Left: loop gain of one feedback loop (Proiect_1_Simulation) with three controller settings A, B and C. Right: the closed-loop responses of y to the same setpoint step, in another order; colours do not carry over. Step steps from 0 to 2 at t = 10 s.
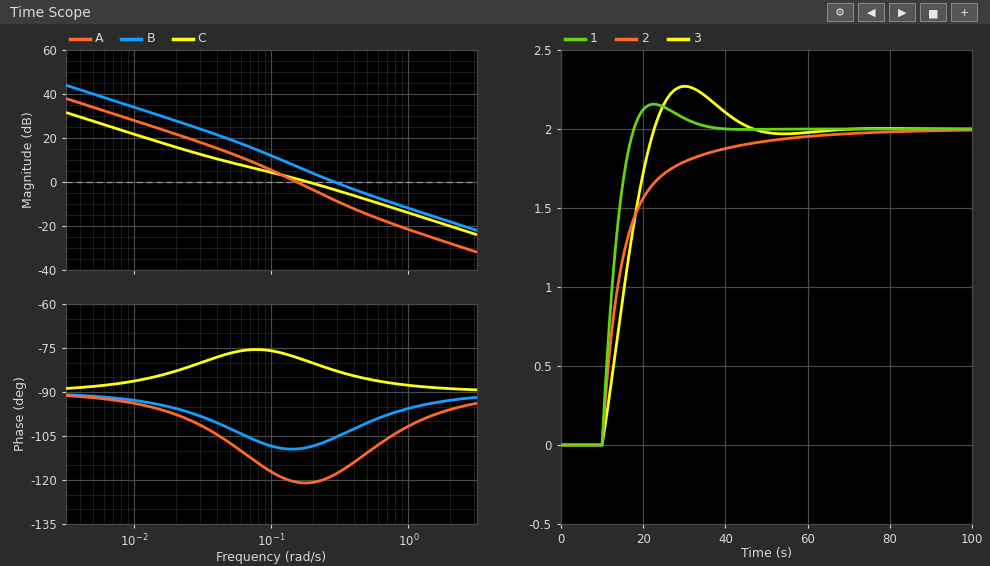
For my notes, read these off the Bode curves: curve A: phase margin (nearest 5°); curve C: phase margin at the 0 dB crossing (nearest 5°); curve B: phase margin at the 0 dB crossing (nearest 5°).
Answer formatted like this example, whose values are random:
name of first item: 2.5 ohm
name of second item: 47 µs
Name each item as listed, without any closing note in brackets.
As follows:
curve A: phase margin: 60°
curve C: phase margin at the 0 dB crossing: 100°
curve B: phase margin at the 0 dB crossing: 75°
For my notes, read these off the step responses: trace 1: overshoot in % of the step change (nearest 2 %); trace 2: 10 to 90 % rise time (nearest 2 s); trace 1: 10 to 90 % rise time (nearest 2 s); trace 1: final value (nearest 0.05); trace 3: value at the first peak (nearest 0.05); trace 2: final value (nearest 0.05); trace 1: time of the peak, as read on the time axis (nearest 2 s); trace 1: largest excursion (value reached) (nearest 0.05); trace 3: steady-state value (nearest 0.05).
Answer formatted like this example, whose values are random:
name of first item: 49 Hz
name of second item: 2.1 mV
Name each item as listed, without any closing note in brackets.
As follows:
trace 1: overshoot in % of the step change: 8 %
trace 2: 10 to 90 % rise time: 20 s
trace 1: 10 to 90 % rise time: 6 s
trace 1: final value: 2.00
trace 3: value at the first peak: 2.25
trace 2: final value: 2.00
trace 1: time of the peak, as read on the time axis: 22 s
trace 1: largest excursion (value reached): 2.15
trace 3: steady-state value: 2.00
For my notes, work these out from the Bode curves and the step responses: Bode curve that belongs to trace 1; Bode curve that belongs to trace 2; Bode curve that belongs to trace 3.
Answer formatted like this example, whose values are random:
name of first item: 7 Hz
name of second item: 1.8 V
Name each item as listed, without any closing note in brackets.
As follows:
Bode curve that belongs to trace 1: B
Bode curve that belongs to trace 2: C
Bode curve that belongs to trace 3: A
